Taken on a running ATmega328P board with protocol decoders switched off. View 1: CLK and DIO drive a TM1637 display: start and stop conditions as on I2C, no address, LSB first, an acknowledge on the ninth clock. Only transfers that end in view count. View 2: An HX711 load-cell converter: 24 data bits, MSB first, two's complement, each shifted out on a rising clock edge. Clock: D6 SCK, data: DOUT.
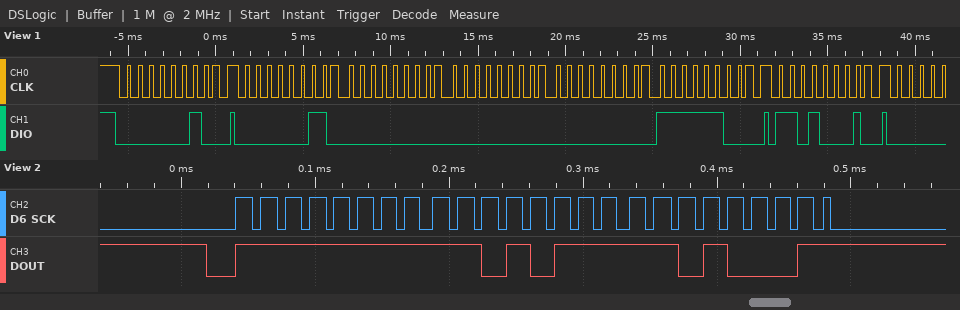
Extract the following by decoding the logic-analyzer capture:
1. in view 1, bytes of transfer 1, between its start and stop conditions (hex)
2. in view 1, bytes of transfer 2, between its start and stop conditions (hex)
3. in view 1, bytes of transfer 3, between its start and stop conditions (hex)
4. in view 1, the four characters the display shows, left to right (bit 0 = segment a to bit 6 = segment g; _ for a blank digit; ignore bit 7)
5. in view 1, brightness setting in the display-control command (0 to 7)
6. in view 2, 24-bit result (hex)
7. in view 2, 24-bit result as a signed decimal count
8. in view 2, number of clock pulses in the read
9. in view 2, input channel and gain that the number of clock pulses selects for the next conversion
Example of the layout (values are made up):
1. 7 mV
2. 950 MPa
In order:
1. 40
2. C0 00 00 00 3F
3. 8B
4. ___0
5. 3
6. 0xFFD7D1
7. -10287
8. 25
9. channel A, gain 128
